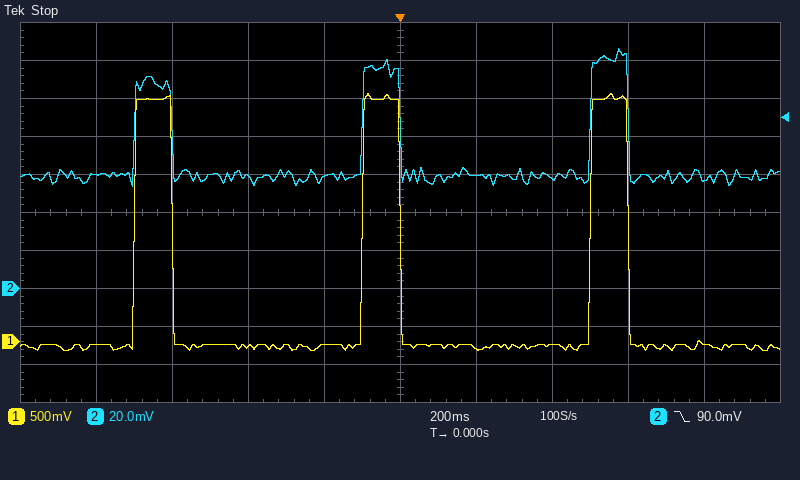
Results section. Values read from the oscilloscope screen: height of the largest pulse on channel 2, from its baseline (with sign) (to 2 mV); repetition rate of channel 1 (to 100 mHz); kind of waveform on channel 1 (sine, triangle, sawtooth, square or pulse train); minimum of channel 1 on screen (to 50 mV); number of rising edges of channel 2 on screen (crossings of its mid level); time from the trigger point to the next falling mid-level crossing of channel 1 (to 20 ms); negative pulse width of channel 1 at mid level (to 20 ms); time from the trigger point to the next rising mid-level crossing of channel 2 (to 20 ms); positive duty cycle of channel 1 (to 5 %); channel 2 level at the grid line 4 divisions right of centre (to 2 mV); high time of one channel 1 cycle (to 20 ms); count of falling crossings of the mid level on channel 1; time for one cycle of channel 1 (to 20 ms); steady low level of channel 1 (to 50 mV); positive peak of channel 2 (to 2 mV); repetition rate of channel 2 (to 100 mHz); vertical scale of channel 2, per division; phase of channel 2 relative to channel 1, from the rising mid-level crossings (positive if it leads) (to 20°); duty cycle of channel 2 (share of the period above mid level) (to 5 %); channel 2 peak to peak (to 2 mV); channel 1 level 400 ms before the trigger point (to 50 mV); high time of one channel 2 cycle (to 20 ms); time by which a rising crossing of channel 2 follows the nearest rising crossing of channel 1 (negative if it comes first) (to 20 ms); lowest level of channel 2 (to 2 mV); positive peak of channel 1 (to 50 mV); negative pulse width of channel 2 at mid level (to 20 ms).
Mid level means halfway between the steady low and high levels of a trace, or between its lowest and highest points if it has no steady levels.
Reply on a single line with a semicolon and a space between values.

+66 mV; 1.7 Hz; pulse train; -100 mV; 3; 600 ms; 500 ms; 500 ms; 15 %; 58 mV; 100 ms; 3; 600 ms; -50 mV; 126 mV; 1.7 Hz; 20 mV; 0°; 15 %; 72 mV; -50 mV; 100 ms; 0 ms; 54 mV; 3.25 V; 500 ms
